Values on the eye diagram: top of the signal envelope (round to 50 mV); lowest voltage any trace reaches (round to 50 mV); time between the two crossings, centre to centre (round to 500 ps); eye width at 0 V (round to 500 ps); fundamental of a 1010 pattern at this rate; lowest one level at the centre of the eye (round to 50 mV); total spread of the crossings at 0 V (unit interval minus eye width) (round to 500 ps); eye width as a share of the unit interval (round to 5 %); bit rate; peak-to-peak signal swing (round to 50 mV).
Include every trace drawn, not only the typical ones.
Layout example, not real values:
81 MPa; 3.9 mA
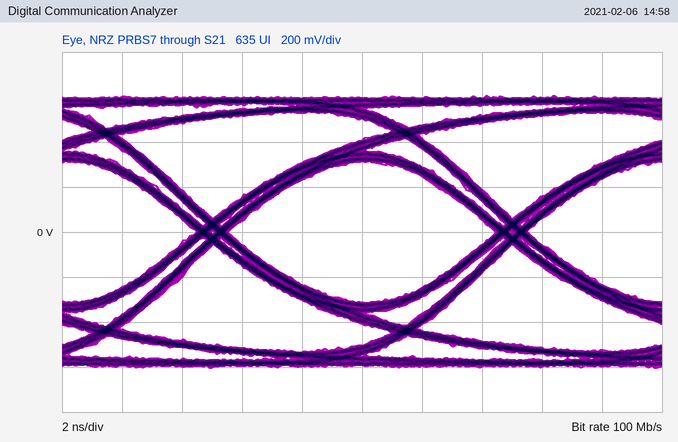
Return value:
600 mV; -600 mV; 10.0 ns; 9.0 ns; 50 MHz; 300 mV; 1.0 ns; 90 %; 100 Mb/s; 1.20 V
